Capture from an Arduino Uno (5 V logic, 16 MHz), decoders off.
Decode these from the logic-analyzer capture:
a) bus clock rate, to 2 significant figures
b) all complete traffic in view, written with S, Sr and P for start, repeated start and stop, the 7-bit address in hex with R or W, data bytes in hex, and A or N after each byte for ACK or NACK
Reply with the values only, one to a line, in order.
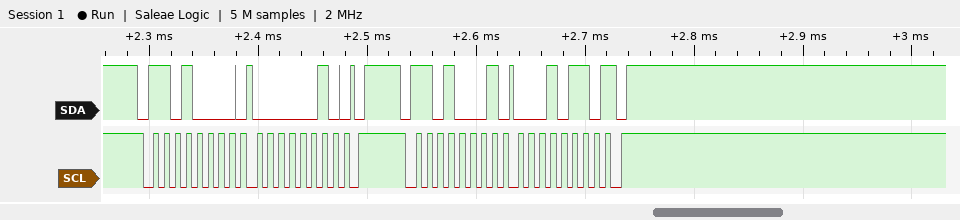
100 kHz
S 68W A 02 A P S 68R A 16 N P
